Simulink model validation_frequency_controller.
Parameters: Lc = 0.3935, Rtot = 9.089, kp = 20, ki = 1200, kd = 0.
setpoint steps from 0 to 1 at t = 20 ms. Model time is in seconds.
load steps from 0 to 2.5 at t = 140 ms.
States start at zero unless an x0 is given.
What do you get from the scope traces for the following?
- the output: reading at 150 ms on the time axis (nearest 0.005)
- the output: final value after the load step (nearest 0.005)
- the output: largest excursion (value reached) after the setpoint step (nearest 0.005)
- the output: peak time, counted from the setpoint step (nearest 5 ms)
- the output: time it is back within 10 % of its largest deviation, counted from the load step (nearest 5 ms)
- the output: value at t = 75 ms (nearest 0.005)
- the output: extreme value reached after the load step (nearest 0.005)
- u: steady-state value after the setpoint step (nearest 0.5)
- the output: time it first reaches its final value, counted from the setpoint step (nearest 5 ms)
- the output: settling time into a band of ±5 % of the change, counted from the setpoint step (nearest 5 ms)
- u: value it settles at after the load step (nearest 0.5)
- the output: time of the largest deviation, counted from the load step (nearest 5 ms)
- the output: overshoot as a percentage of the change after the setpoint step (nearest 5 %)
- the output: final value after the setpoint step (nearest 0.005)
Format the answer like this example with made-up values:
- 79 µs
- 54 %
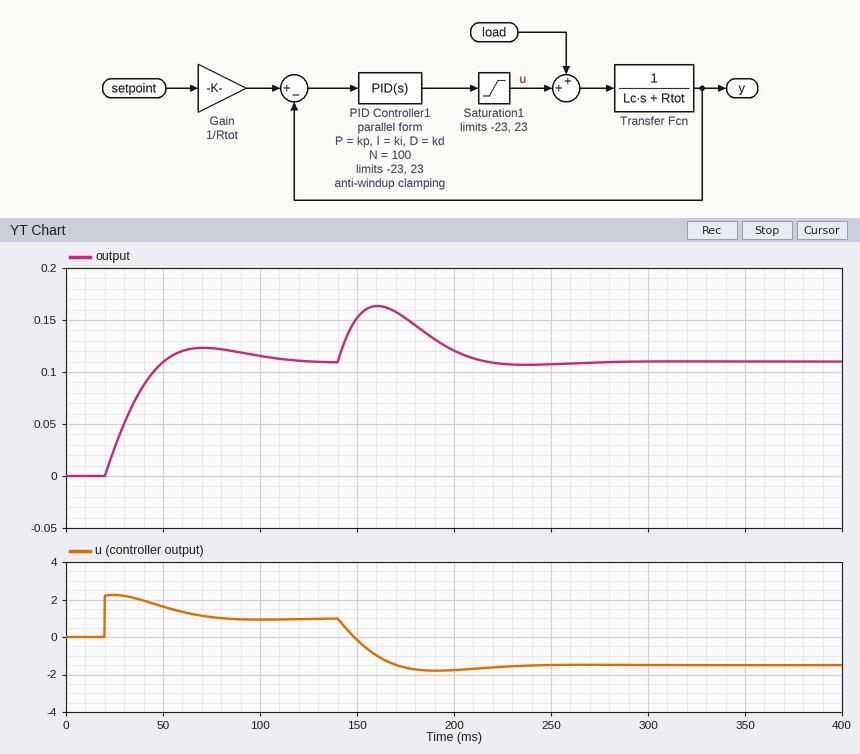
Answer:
- 0.150
- 0.110
- 0.125
- 50 ms
- 65 ms
- 0.125
- 0.165
- 1.0
- 30 ms
- 80 ms
- -1.5
- 20 ms
- 10 %
- 0.110
